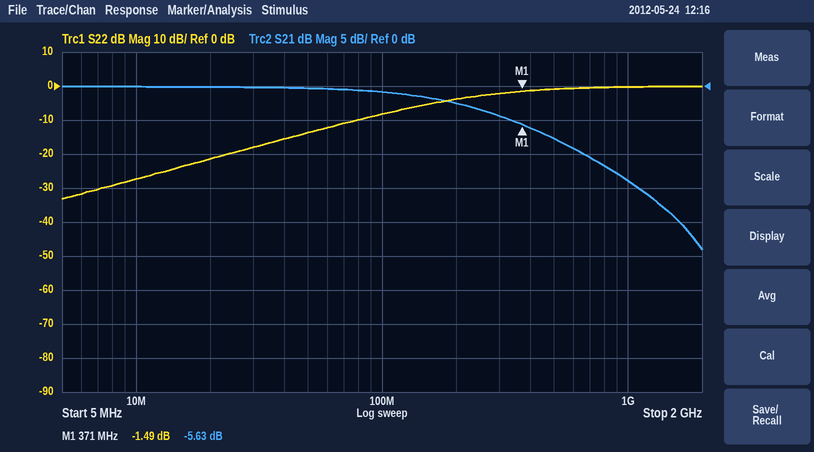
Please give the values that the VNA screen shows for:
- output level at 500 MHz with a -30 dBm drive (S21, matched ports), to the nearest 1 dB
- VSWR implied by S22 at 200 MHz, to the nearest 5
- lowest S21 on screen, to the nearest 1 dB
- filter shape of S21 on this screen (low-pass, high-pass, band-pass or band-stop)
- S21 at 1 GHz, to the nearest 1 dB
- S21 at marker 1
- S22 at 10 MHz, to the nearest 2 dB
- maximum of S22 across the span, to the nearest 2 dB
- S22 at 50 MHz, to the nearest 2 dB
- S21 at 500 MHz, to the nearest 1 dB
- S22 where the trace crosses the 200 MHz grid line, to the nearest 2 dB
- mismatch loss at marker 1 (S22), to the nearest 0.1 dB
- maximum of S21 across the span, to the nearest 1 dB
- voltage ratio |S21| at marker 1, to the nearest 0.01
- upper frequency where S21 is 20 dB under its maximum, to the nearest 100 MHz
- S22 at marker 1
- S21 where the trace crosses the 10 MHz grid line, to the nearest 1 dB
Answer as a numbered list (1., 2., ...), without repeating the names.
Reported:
1. -38 dBm
2. 5
3. -24 dB
4. low-pass
5. -14 dB
6. -5.63 dB
7. -28 dB
8. 0 dB
9. -14 dB
10. -8 dB
11. -4 dB
12. 5.4 dB
13. 0 dB
14. 0.52
15. 1.6 GHz
16. -1.49 dB
17. 0 dB
